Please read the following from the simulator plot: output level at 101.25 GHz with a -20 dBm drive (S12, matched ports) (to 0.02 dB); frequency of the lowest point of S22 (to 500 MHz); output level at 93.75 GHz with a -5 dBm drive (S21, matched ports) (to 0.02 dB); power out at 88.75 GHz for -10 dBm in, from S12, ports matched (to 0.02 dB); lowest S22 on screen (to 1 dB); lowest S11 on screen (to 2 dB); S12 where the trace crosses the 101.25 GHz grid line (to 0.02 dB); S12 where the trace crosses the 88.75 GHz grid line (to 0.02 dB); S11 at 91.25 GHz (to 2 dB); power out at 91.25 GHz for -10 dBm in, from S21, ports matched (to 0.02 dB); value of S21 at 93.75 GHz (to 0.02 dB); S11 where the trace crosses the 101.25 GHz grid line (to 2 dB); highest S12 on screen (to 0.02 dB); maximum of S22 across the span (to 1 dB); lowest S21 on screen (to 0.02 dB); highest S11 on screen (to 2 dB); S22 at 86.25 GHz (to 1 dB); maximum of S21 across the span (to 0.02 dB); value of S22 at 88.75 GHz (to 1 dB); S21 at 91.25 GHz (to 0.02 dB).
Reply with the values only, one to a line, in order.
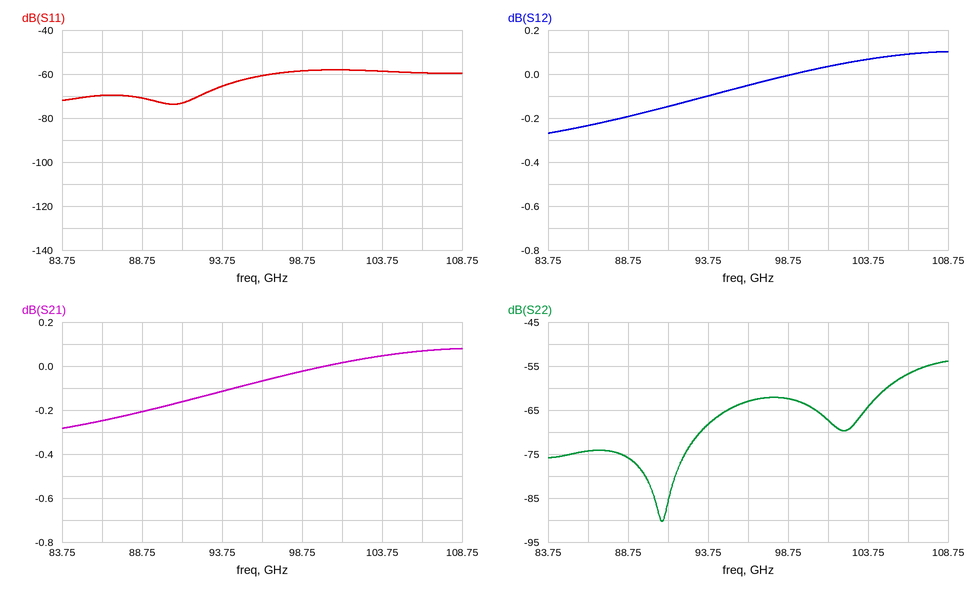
-19.96 dBm
91.0 GHz
-5.12 dBm
-10.20 dBm
-90 dB
-74 dB
0.04 dB
-0.20 dB
-74 dB
-10.16 dBm
-0.12 dB
-58 dB
0.10 dB
-54 dB
-0.28 dB
-58 dB
-74 dB
0.08 dB
-76 dB
-0.16 dB
